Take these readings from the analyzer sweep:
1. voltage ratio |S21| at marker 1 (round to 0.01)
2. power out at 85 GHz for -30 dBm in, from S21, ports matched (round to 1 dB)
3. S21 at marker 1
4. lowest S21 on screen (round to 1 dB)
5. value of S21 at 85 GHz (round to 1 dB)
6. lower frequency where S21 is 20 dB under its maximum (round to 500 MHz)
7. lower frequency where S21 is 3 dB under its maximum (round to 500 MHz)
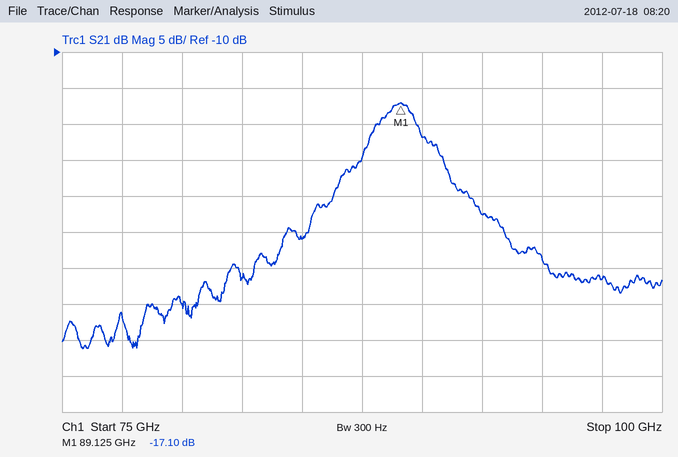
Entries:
0.14
-66 dBm
-17.10 dB
-51 dB
-36 dB
84.0 GHz
88.0 GHz
